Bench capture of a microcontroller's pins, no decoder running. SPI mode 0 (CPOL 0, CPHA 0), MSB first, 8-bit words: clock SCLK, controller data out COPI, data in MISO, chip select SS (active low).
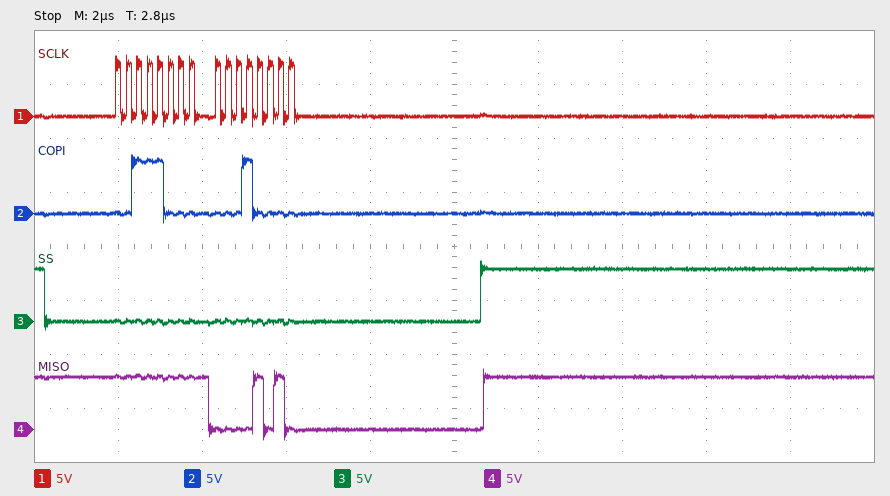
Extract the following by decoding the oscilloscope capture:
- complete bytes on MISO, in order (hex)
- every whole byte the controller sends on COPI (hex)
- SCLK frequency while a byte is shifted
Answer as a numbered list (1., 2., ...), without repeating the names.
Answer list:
1. FF 0A
2. 38 10
3. 4 MHz
